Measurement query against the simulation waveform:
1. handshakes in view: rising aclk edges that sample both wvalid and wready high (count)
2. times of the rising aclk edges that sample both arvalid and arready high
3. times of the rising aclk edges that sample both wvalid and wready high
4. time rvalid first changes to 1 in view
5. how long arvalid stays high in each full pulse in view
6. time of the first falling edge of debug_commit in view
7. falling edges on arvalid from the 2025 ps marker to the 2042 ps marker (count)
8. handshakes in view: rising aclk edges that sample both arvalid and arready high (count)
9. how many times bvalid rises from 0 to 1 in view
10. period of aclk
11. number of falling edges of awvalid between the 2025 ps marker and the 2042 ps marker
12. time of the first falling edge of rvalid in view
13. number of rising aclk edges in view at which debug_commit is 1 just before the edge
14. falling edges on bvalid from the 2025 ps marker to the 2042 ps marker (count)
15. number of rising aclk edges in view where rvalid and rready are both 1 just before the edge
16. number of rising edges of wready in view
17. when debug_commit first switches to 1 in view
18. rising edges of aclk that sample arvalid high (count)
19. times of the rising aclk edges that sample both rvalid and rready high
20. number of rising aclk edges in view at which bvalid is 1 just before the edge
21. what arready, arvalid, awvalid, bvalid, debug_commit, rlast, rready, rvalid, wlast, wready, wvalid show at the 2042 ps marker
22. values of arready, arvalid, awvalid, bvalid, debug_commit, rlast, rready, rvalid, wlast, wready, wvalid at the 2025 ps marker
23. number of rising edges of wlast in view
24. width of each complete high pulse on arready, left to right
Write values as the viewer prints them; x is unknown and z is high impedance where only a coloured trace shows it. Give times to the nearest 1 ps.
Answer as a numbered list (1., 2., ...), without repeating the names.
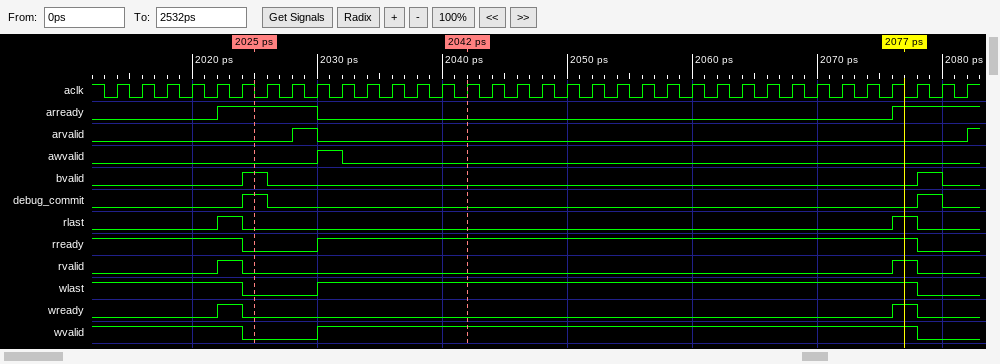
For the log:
1. 2
2. 2030 ps
3. 2024 ps, 2078 ps
4. 2022 ps
5. 2 ps
6. 2026 ps
7. 1
8. 1
9. 2
10. 2 ps
11. 1
12. 2024 ps
13. 2
14. 1
15. 2
16. 2
17. 2024 ps
18. 1
19. 2024 ps, 2078 ps
20. 2
21. arready=0, arvalid=0, awvalid=0, bvalid=0, debug_commit=0, rlast=0, rready=1, rvalid=0, wlast=1, wready=0, wvalid=1
22. arready=1, arvalid=0, awvalid=0, bvalid=1, debug_commit=1, rlast=0, rready=0, rvalid=0, wlast=0, wready=0, wvalid=0
23. 1
24. 8 ps
